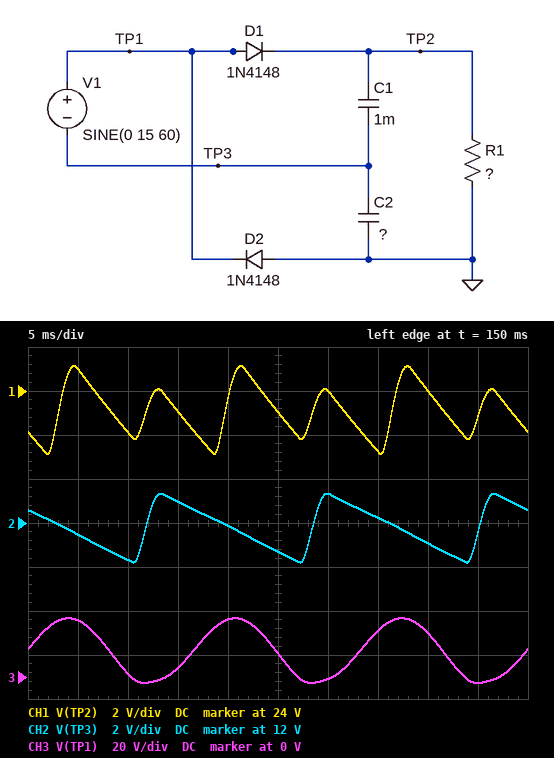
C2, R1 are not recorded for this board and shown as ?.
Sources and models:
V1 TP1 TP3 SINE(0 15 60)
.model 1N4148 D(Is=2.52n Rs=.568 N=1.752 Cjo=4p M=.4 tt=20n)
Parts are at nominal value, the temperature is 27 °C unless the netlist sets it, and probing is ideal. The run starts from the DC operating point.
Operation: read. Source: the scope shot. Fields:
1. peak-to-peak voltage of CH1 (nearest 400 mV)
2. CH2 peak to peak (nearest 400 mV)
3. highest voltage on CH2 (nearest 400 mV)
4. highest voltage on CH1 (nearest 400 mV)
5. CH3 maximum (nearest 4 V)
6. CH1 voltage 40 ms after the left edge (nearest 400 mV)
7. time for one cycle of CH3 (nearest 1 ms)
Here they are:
4.0 V
3.2 V
13.2 V
25.2 V
28 V
24.0 V
17 ms
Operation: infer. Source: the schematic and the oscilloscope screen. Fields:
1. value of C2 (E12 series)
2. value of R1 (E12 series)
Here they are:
1.5 mF
68 Ω
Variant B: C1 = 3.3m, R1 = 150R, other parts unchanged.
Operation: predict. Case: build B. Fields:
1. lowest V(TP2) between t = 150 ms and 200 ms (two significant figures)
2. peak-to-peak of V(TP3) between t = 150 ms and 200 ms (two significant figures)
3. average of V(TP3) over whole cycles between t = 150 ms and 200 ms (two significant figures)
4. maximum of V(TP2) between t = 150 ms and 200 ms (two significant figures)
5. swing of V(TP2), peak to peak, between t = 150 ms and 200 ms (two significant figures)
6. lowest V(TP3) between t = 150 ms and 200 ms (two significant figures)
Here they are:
25 V
1.6 V
13 V
26 V
1.5 V
12 V
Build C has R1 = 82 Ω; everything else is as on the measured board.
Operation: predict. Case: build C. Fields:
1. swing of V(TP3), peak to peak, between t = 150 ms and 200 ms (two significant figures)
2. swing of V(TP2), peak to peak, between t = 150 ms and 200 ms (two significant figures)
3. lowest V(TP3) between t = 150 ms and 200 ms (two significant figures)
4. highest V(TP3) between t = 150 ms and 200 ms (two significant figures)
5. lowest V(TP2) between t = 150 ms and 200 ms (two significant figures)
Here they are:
2.7 V
3.5 V
11 V
13 V
22 V
